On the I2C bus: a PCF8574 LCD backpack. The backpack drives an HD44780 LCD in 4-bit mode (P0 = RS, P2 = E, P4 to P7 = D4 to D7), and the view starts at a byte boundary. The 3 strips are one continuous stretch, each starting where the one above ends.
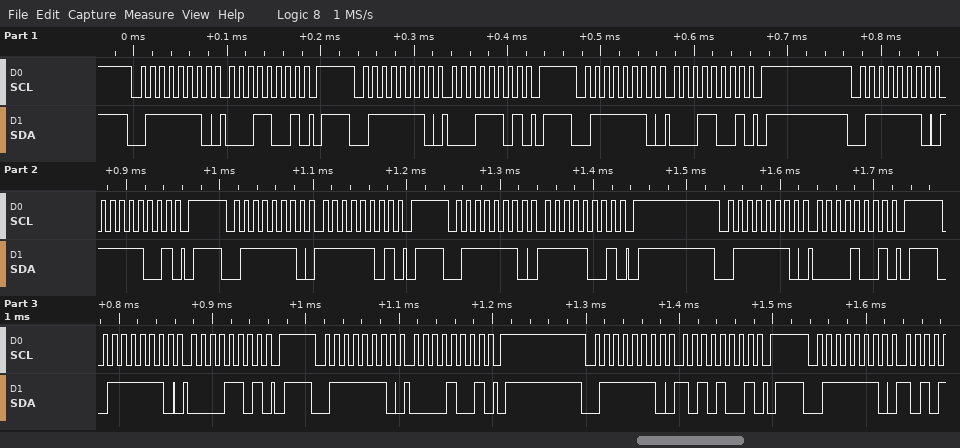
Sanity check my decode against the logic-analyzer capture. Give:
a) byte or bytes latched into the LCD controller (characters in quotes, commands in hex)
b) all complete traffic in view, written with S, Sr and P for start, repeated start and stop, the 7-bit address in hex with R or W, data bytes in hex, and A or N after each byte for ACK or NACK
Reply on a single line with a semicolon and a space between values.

data 0x1F; S 3FW A 19 A P S 3FW A 1D A P S 3FW A 19 A P S 3FW A F9 A P S 3FW A FD A P S 3FW A F9 A P S 3FW A 09 A P S 3FW A 0D A P S 3FW A 09 A P S 3FW A A9 A P S 3FW A
